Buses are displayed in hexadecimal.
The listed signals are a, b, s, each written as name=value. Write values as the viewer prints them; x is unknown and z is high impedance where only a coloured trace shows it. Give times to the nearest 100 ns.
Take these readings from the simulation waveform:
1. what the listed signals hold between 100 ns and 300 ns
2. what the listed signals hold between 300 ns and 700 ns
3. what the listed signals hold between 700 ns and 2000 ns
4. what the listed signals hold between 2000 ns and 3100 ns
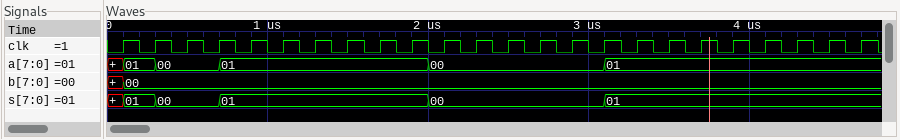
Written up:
a=01, b=00, s=01
a=00, b=00, s=00
a=01, b=00, s=01
a=00, b=00, s=00
